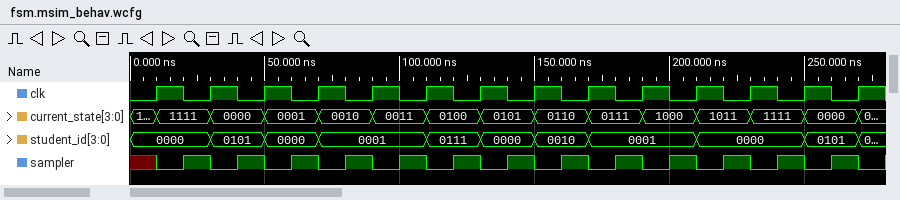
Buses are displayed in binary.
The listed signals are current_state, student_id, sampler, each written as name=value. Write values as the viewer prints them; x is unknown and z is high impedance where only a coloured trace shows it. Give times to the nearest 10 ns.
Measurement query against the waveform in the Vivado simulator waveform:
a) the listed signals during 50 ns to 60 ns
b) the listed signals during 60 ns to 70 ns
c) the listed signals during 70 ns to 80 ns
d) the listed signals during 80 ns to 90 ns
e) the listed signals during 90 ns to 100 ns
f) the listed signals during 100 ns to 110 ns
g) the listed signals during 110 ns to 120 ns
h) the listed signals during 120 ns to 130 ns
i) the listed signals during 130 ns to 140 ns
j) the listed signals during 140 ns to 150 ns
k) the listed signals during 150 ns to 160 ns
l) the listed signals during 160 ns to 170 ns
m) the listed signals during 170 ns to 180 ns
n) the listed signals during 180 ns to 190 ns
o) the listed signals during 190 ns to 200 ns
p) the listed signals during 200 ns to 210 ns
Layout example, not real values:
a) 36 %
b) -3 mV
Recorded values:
a) current_state=0001, student_id=0000, sampler=0
b) current_state=0001, student_id=0000, sampler=1
c) current_state=0010, student_id=0001, sampler=0
d) current_state=0010, student_id=0001, sampler=1
e) current_state=0011, student_id=0001, sampler=0
f) current_state=0011, student_id=0001, sampler=1
g) current_state=0100, student_id=0111, sampler=0
h) current_state=0100, student_id=0111, sampler=1
i) current_state=0101, student_id=0000, sampler=0
j) current_state=0101, student_id=0000, sampler=1
k) current_state=0110, student_id=0010, sampler=0
l) current_state=0110, student_id=0010, sampler=1
m) current_state=0111, student_id=0001, sampler=0
n) current_state=0111, student_id=0001, sampler=1
o) current_state=1000, student_id=0001, sampler=0
p) current_state=1000, student_id=0001, sampler=1
